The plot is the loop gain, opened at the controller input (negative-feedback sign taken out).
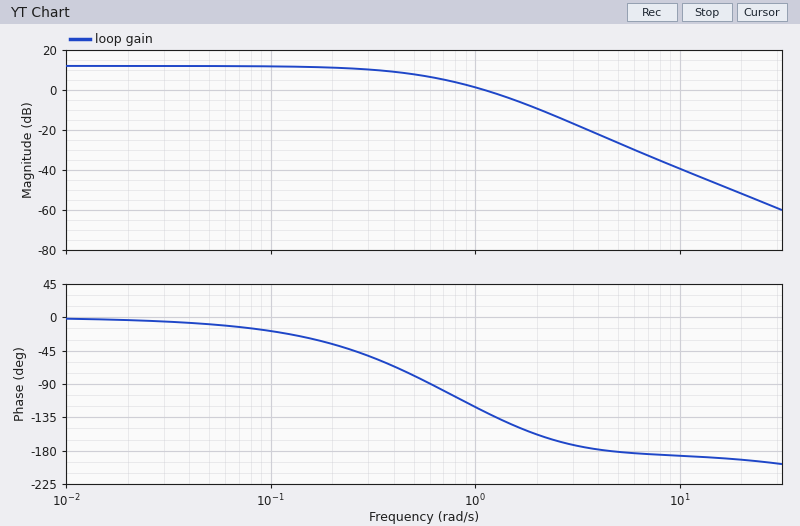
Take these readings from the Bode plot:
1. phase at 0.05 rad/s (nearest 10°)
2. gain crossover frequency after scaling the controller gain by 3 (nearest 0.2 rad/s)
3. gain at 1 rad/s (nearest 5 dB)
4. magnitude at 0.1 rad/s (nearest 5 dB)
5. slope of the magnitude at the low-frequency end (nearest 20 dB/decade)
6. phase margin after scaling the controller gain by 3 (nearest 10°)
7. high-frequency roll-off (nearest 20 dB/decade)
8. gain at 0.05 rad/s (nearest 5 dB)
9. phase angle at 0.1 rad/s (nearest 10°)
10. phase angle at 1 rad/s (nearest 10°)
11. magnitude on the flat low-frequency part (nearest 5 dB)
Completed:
-10°
2.0 rad/s
0 dB
10 dB
0 dB/decade
20°
-40 dB/decade
10 dB
-20°
-120°
10 dB
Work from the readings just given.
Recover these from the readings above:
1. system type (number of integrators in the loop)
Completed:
0
